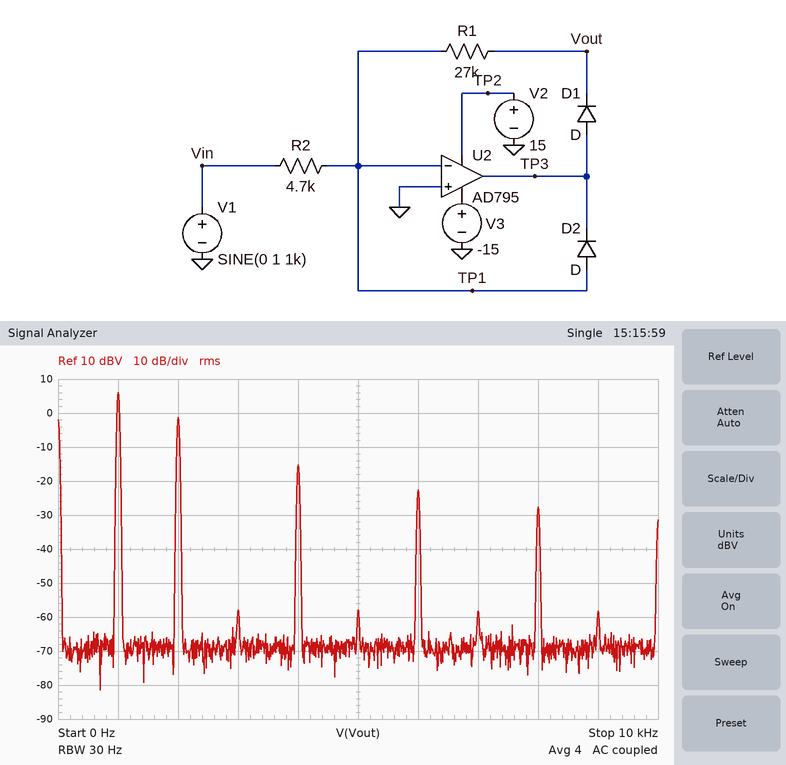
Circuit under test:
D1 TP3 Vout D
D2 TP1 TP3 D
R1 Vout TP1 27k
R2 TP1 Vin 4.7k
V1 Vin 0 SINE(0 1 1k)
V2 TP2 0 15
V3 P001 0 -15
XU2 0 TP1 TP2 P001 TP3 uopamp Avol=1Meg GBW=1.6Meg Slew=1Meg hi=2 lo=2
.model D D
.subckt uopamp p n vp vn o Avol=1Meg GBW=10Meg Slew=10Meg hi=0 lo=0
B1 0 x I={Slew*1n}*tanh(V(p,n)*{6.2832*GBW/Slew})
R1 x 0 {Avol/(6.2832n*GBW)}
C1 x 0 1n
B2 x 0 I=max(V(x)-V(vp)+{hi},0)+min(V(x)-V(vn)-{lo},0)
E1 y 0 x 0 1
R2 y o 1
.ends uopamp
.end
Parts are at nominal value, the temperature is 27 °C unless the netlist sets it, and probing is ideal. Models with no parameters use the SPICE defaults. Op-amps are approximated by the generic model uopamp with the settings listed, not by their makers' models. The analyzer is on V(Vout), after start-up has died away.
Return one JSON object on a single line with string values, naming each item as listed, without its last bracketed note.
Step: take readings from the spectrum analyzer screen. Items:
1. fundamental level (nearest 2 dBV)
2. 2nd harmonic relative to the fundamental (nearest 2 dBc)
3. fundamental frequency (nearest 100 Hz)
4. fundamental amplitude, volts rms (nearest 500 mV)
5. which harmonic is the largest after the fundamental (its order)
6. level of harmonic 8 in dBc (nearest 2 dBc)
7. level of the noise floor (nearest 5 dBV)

{"fundamental level": "6 dBV", "2nd harmonic relative to the fundamental": "-8 dBc", "fundamental frequency": "1.0 kHz", "fundamental amplitude, volts rms": "2.0 V", "which harmonic is the largest after the fundamental": "2", "level of harmonic 8 in dBc": "-34 dBc", "level of the noise floor": "-70 dBV"}
